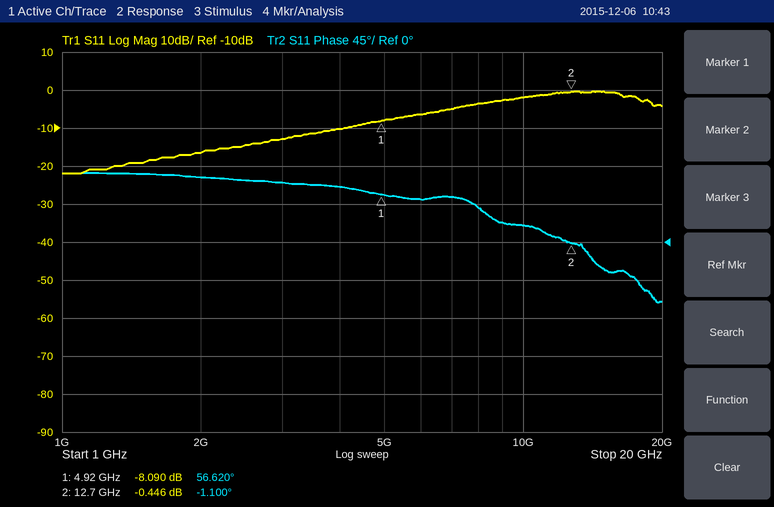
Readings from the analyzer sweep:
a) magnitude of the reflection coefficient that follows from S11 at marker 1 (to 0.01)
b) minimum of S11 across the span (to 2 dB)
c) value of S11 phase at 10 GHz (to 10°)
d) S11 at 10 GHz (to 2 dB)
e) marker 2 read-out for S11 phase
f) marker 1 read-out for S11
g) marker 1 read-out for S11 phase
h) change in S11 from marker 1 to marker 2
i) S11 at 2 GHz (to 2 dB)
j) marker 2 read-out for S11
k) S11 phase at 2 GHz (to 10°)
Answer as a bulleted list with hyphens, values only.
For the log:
- 0.39
- -22 dB
- 20°
- -2 dB
- -1.100°
- -8.090 dB
- 56.620°
- 7.644 dB
- -16 dB
- -0.446 dB
- 80°
